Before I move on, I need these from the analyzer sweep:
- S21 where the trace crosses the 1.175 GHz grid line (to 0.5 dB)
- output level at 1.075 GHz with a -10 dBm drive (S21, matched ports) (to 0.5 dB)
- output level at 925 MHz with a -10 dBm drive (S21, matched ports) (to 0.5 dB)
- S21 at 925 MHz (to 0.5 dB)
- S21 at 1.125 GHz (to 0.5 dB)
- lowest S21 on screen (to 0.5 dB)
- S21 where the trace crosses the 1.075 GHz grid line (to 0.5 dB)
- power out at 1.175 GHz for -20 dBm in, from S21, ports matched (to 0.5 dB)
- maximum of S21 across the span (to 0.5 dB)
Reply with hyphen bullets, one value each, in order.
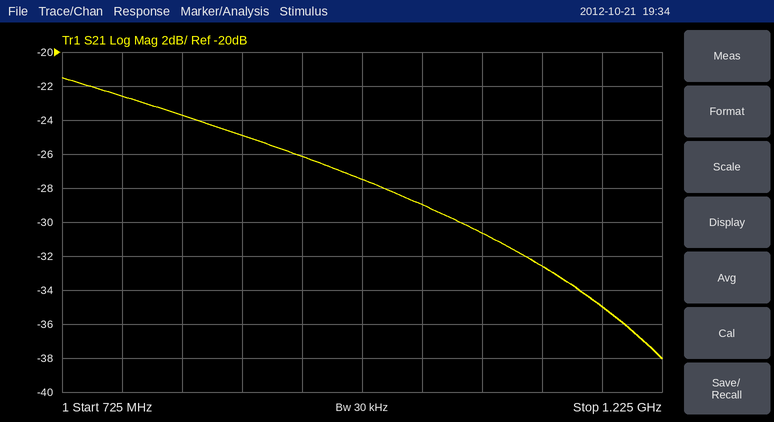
- -35.0 dB
- -40.5 dBm
- -36.0 dBm
- -26.0 dB
- -32.5 dB
- -38.0 dB
- -30.5 dB
- -55.0 dBm
- -21.5 dB
